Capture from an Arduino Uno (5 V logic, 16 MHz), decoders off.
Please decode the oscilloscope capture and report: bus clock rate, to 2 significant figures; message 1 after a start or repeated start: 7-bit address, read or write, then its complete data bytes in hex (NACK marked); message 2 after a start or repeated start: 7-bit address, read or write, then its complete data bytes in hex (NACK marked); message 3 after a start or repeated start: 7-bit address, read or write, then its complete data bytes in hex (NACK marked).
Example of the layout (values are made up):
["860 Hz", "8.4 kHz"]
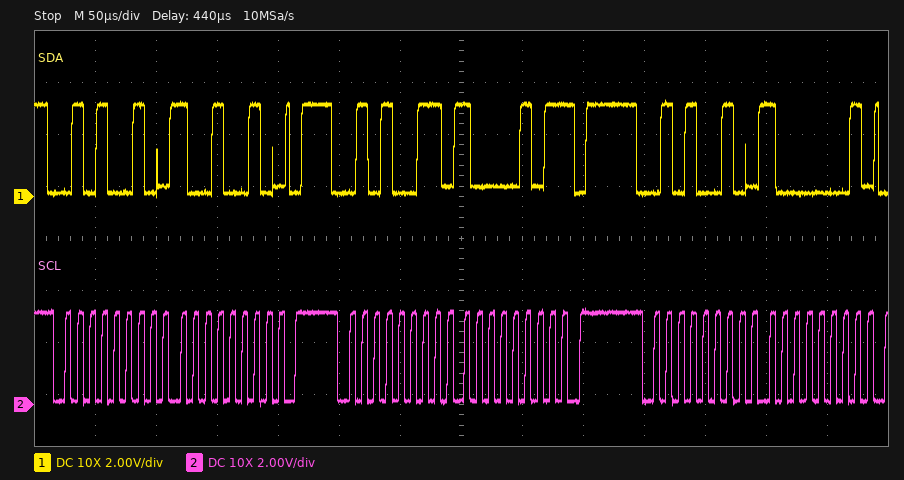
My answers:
["100 kHz", "0x29 write: 92", "0x29 read: 85 NACK", "0x29 write: 81"]
